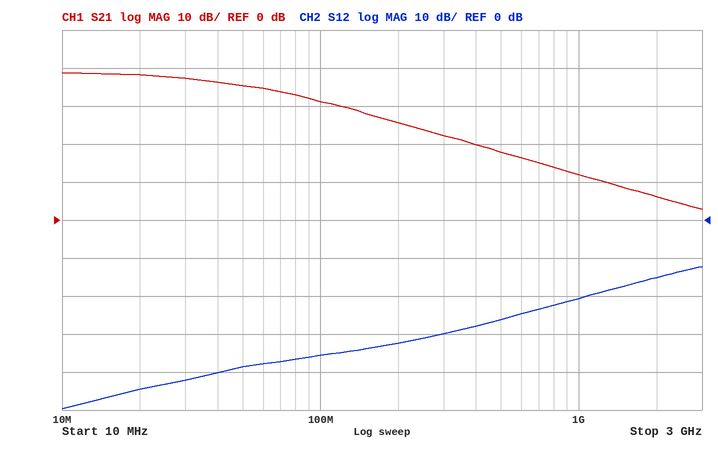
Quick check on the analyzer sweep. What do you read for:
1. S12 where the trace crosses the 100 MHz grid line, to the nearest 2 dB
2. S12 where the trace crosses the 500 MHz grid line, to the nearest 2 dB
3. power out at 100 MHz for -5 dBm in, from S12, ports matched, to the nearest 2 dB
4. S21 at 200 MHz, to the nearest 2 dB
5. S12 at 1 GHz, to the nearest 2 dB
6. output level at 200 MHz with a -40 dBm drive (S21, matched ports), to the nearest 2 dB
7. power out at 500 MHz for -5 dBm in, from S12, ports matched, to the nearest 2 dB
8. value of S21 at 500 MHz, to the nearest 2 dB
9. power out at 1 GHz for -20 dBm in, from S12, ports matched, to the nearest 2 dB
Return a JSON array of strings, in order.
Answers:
["-36 dB", "-26 dB", "-40 dBm", "26 dB", "-20 dB", "-14 dBm", "-32 dBm", "18 dB", "-40 dBm"]
